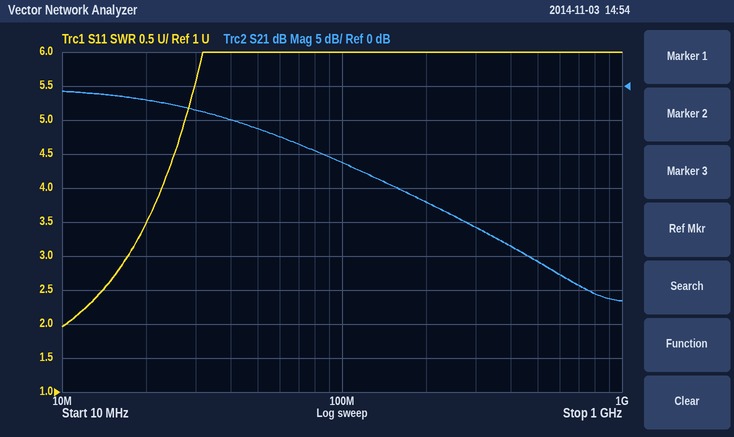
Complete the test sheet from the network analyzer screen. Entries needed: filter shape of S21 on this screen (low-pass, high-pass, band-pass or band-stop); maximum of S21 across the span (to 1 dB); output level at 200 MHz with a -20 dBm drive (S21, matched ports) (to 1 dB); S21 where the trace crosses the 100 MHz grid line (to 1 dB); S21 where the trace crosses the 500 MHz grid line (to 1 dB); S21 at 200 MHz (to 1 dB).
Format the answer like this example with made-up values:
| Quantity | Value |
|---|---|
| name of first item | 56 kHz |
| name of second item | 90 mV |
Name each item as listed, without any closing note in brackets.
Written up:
| Quantity | Value |
|---|---|
| filter shape of S21 on this screen | low-pass |
| maximum of S21 across the span | -1 dB |
| output level at 200 MHz with a -20 dBm drive (S21, matched ports) | -37 dBm |
| S21 where the trace crosses the 100 MHz grid line | -11 dB |
| S21 where the trace crosses the 500 MHz grid line | -26 dB |
| S21 at 200 MHz | -17 dB |
